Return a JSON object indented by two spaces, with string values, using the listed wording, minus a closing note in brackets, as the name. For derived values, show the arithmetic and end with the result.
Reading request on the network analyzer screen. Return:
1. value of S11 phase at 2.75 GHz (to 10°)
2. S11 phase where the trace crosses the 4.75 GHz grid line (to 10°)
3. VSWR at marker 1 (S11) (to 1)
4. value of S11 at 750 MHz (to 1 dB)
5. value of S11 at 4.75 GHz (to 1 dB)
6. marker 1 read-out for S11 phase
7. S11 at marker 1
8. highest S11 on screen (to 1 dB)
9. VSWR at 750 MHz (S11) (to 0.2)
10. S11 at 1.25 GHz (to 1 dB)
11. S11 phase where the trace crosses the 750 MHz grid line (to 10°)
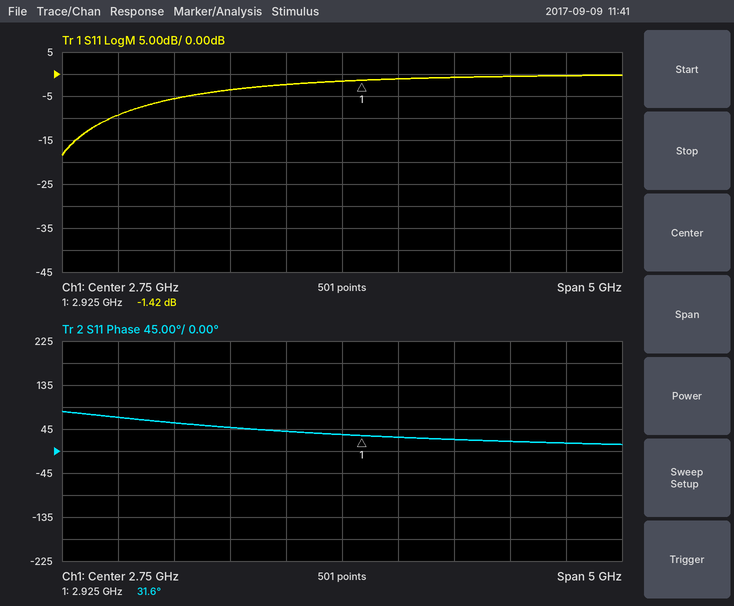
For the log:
{
  "value of S11 phase at 2.75 GHz": "30°",
  "S11 phase where the trace crosses the 4.75 GHz grid line": "20°",
  "VSWR at marker 1 (S11)": "(1 + 0.8492)/(1 − 0.8492) ≈ 12",
  "value of S11 at 750 MHz": "-9 dB",
  "value of S11 at 4.75 GHz": "0 dB",
  "marker 1 read-out for S11 phase": "31.6°",
  "S11 at marker 1": "-1.42 dB",
  "highest S11 on screen": "0 dB",
  "VSWR at 750 MHz (S11)": "|Γ| = 10^(-9/20) = 0.3548; VSWR = (1 + 0.3548)/(1 − 0.3548) ≈ 2.10, so 2.0 to the nearest 0.2",
  "S11 at 1.25 GHz": "-6 dB",
  "S11 phase where the trace crosses the 750 MHz grid line": "70°"
}
